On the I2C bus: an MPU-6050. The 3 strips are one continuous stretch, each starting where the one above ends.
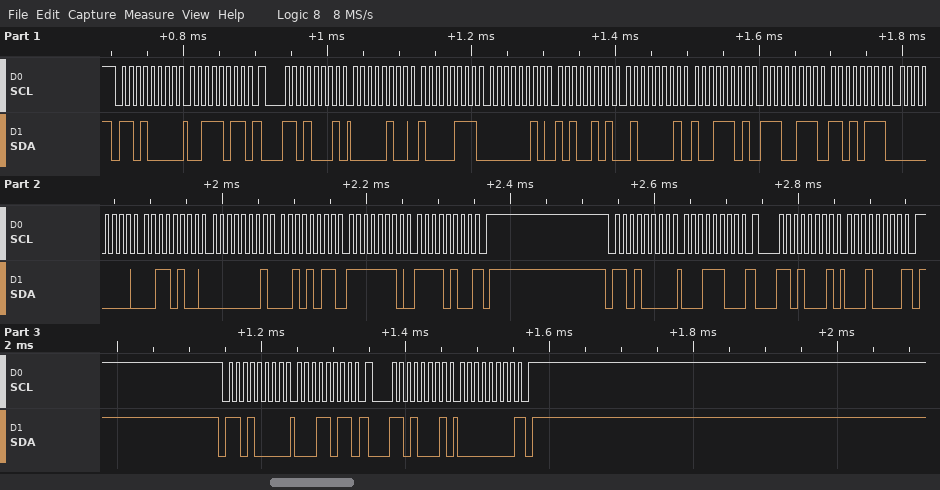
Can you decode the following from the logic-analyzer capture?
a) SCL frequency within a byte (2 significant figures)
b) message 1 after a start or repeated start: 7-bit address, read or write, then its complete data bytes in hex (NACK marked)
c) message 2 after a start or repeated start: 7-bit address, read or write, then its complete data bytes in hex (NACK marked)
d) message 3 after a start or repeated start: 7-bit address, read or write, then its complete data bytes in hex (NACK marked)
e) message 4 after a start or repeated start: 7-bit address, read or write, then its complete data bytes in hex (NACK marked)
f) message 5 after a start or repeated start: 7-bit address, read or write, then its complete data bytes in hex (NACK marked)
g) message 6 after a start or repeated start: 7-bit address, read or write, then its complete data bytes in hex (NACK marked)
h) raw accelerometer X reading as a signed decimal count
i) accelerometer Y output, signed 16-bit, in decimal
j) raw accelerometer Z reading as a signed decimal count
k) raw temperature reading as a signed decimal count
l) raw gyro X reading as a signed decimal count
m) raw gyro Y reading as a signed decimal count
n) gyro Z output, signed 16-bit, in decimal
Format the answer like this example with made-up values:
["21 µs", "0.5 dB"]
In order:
["100 kHz", "0x68 write: 3B", "0x68 read: 04 87 02 A5 41 9D E7 D7 00 34 01 2B FE F4 NACK", "0x68 write: 1C", "0x68 read: 10 NACK", "0x68 write: 1B", "0x68 read: 00 NACK", "1159", "677", "16797", "-6185", "52", "299", "-268"]
